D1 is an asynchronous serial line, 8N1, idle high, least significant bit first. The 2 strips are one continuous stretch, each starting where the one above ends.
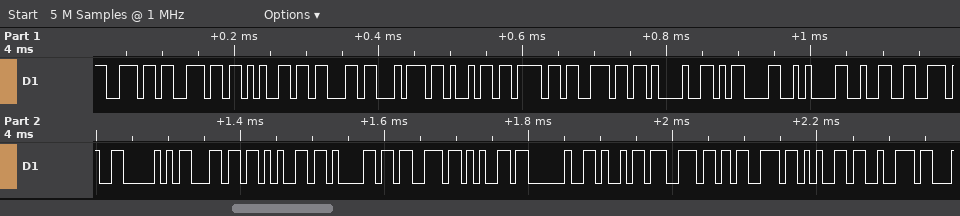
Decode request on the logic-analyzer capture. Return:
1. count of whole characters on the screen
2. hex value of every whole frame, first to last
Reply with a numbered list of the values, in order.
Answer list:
1. 25
2. 0x6E 0x6E 0x65 0x63 0x74 0x69 0x6F 0x6E 0x21 0x0D 0x0A 0x32 0x2E 0x50 0x6C 0x65 0x61 0x73 0x65 0x20 0x69 0x6E 0x73 0x65 0x72
